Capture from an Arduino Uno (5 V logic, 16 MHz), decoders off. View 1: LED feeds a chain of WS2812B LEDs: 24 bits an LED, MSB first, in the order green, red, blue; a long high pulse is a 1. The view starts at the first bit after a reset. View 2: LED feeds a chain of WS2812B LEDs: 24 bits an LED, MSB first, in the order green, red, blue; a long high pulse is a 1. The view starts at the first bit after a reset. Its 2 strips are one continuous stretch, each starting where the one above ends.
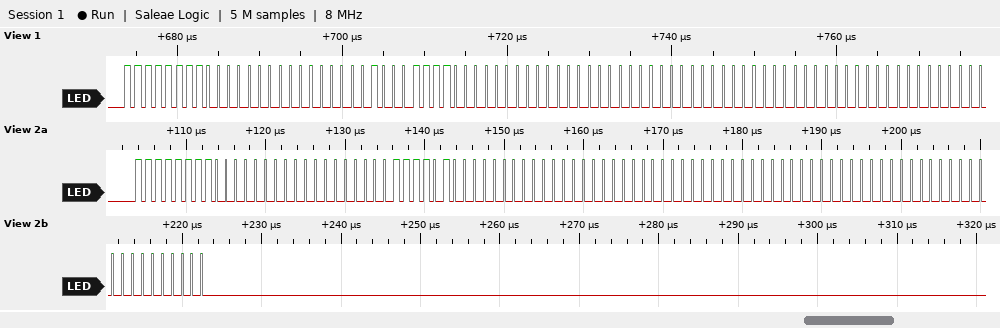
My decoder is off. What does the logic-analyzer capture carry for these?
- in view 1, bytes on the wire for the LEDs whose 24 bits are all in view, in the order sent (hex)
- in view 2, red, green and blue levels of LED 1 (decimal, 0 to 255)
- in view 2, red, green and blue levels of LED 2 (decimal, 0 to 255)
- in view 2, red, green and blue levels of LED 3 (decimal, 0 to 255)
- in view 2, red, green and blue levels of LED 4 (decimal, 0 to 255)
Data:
FF 00 00 8F 00 00 00 00 00
0, 255, 0
0, 61, 0
0, 0, 0
0, 0, 0
